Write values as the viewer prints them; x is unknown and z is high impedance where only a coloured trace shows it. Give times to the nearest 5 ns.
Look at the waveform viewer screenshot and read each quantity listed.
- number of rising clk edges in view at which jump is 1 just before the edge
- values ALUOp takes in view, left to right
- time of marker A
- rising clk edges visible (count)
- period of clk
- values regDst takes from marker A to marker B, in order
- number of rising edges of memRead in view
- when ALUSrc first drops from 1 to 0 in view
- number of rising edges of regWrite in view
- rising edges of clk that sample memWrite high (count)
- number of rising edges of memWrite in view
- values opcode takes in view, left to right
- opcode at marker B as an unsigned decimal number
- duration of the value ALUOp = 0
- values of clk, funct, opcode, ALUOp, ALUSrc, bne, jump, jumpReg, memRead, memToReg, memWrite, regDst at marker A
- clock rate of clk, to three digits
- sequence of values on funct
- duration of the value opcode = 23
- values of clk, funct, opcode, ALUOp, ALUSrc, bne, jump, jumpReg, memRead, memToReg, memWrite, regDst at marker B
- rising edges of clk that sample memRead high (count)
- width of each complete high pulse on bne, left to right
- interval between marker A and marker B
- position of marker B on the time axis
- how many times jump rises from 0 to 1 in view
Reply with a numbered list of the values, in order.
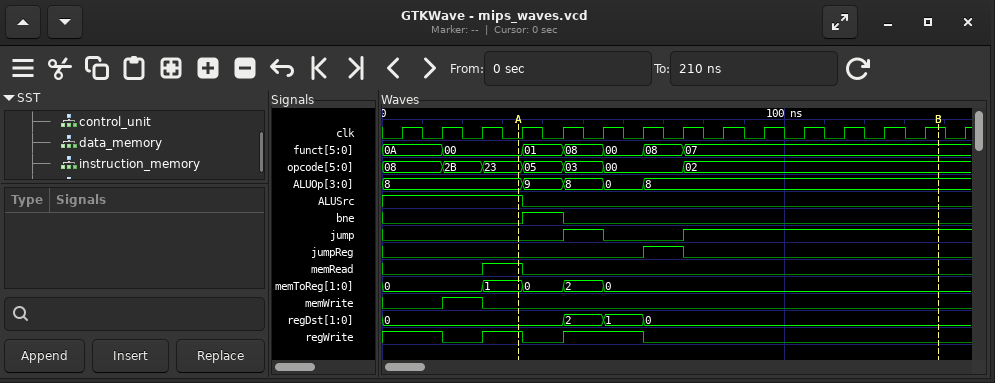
1. 8
2. 8, 9, 8, 0, 8
3. 35 ns
4. 15
5. 10 ns
6. 0, 2, 1, 0
7. 1
8. 35 ns
9. 2
10. 1
11. 1
12. 08, 2B, 23, 05, 03, 00, 02
13. 2
14. 10 ns
15. clk=0, funct=00, opcode=23, ALUOp=8, ALUSrc=1, bne=0, jump=0, jumpReg=0, memRead=1, memToReg=1, memWrite=0, regDst=0
16. 100 MHz
17. 0A, 00, 01, 08, 00, 08, 07
18. 10 ns
19. clk=1, funct=07, opcode=02, ALUOp=8, ALUSrc=0, bne=0, jump=1, jumpReg=0, memRead=0, memToReg=0, memWrite=0, regDst=0
20. 1
21. 10 ns
22. 105 ns
23. 140 ns
24. 2
